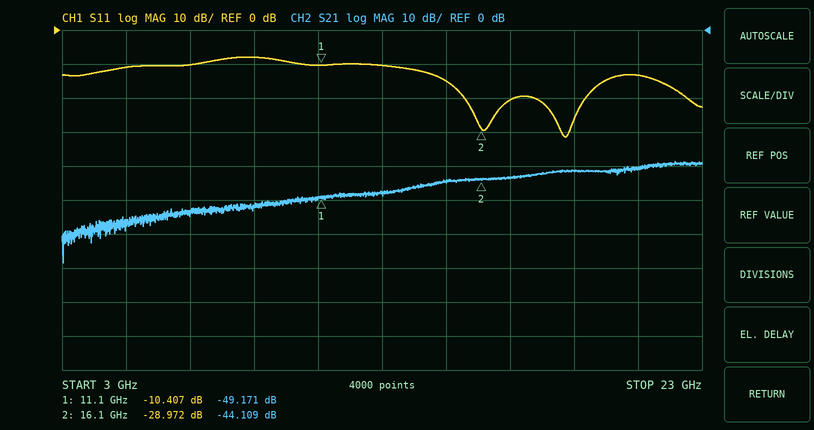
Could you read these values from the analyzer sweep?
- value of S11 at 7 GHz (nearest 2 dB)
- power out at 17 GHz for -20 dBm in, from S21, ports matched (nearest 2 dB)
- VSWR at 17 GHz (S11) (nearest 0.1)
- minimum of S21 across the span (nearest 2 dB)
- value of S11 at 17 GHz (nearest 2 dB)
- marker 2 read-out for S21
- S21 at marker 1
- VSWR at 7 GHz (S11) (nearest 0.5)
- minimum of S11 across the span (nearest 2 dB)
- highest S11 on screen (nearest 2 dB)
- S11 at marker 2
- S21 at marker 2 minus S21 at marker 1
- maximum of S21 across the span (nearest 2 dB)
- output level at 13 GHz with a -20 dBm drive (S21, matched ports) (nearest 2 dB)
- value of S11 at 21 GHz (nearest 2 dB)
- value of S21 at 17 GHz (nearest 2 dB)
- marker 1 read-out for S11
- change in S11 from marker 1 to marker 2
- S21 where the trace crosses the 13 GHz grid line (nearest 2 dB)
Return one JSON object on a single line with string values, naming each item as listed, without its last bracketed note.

{"value of S11 at 7 GHz": "-10 dB", "power out at 17 GHz for -20 dBm in, from S21, ports matched": "-64 dBm", "VSWR at 17 GHz (S11)": "1.2", "minimum of S21 across the span": "-68 dB", "value of S11 at 17 GHz": "-20 dB", "marker 2 read-out for S21": "-44.109 dB", "S21 at marker 1": "-49.171 dB", "VSWR at 7 GHz (S11)": "2.0", "minimum of S11 across the span": "-32 dB", "highest S11 on screen": "-8 dB", "S11 at marker 2": "-28.972 dB", "S21 at marker 2 minus S21 at marker 1": "5.062 dB", "maximum of S21 across the span": "-38 dB", "output level at 13 GHz with a -20 dBm drive (S21, matched ports)": "-68 dBm", "value of S11 at 21 GHz": "-14 dB", "value of S21 at 17 GHz": "-44 dB", "marker 1 read-out for S11": "-10.407 dB", "change in S11 from marker 1 to marker 2": "-18.565 dB", "S21 where the trace crosses the 13 GHz grid line": "-48 dB"}
